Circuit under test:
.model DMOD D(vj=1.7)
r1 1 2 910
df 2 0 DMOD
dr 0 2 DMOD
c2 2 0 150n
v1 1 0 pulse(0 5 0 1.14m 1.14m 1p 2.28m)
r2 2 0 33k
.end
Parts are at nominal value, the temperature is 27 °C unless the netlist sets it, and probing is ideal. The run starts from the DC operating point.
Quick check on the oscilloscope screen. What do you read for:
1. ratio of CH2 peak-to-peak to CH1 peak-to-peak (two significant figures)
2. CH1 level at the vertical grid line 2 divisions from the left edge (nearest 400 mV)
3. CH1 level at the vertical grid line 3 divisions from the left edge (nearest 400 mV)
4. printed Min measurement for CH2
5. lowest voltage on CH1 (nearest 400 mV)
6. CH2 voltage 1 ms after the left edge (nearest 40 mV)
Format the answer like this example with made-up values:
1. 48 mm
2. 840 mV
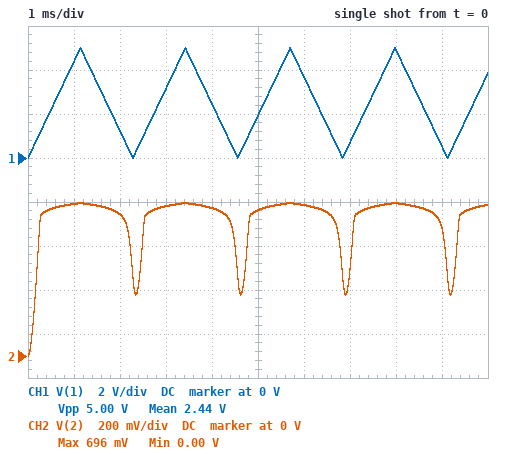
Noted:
1. 0.14
2. 1.2 V
3. 3.2 V
4. 0.00 V
5. 0 V
6. 680 mV
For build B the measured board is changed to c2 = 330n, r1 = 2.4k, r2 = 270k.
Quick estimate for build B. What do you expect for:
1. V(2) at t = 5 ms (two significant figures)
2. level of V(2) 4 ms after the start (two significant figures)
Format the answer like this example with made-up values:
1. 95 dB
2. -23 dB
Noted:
1. 640 mV
2. 650 mV
